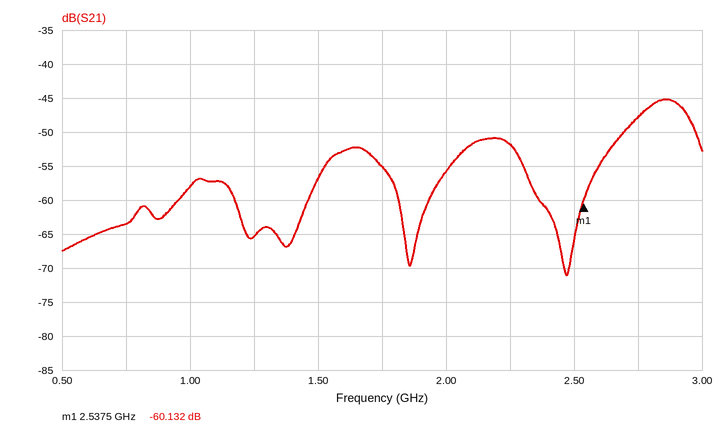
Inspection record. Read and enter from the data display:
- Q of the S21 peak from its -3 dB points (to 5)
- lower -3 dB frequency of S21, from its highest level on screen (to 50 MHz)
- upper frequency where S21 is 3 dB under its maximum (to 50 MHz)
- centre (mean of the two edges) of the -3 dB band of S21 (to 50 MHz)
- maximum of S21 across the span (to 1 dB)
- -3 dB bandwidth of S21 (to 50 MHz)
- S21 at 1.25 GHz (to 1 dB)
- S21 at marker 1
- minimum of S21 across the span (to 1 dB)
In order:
15
2.75 GHz
2.95 GHz
2.85 GHz
-45 dB
200 MHz
-65 dB
-60.132 dB
-71 dB
